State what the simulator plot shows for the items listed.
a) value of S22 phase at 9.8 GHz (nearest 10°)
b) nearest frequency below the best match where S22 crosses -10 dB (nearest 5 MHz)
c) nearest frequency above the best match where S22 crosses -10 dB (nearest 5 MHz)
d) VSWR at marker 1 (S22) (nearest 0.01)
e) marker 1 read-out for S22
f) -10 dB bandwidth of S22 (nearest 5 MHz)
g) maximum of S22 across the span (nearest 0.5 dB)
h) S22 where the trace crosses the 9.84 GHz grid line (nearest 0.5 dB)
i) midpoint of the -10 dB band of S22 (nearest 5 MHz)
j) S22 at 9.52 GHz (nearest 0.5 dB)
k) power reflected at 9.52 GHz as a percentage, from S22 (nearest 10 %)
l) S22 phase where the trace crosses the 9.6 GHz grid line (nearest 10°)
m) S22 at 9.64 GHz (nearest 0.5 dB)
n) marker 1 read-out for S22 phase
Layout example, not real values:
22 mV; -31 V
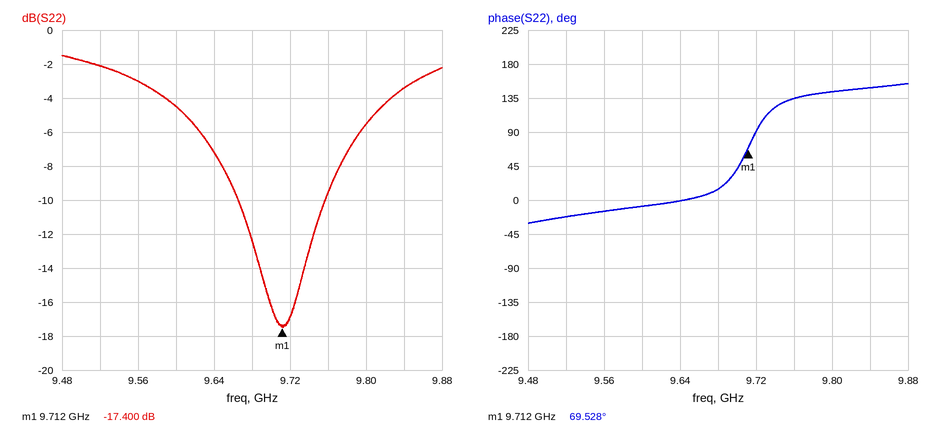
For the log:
140°; 9.665 GHz; 9.755 GHz; 1.31; -17.400 dB; 90 MHz; -1.5 dB; -3.5 dB; 9.710 GHz; -2.0 dB; 60 %; -10°; -7.0 dB; 69.528°
